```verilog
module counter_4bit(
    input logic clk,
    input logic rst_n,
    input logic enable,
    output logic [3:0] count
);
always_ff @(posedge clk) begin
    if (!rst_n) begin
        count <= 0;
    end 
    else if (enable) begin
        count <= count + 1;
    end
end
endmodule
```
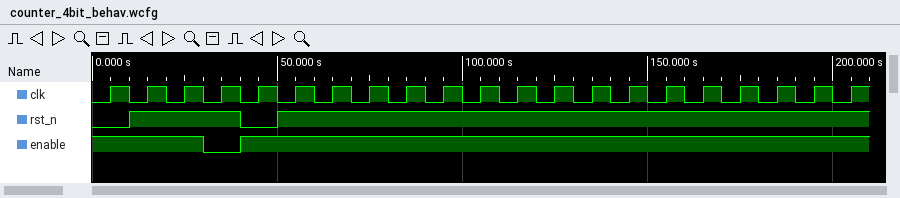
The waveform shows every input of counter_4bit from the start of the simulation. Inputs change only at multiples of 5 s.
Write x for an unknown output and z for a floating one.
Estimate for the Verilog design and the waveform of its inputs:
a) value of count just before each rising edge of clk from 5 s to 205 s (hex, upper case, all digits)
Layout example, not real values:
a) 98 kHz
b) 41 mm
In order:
a) x, 0, 1, 2, 2, 0, 1, 2, 3, 4, 5, 6, 7, 8, 9, A, B, C, D, E, F
